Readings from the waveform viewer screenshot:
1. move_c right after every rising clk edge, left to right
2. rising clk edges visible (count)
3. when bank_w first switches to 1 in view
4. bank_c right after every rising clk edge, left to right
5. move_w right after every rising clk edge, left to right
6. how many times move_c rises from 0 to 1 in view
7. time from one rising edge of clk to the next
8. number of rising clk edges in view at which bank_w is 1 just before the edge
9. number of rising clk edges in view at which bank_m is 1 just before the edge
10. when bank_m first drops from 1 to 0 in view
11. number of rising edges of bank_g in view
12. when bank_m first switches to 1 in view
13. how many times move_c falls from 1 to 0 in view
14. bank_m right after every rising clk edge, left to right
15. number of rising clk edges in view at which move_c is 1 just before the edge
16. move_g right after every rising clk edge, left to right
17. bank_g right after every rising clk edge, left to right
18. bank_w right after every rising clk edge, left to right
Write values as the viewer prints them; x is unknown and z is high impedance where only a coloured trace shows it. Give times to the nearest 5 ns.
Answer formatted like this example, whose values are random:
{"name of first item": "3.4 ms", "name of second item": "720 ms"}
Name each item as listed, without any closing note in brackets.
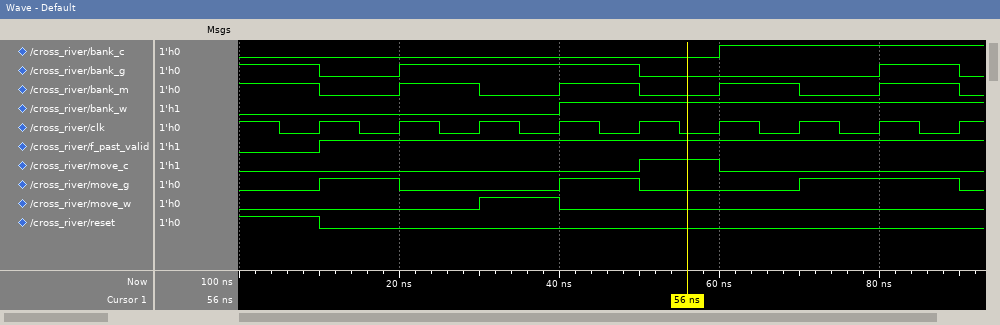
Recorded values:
{"move_c right after every rising clk edge, left to right": "0 0 0 0 1 0 0 0 0", "rising clk edges visible": "9", "when bank_w first switches to 1 in view": "40 ns", "bank_c right after every rising clk edge, left to right": "0 0 0 0 0 1 1 1 1", "move_w right after every rising clk edge, left to right": "0 0 1 0 0 0 0 0 0", "how many times move_c rises from 0 to 1 in view": "1", "time from one rising edge of clk to the next": "10 ns", "number of rising clk edges in view at which bank_w is 1 just before the edge": "5", "number of rising clk edges in view at which bank_m is 1 just before the edge": "5", "when bank_m first drops from 1 to 0 in view": "10 ns", "number of rising edges of bank_g in view": "2", "when bank_m first switches to 1 in view": "20 ns", "how many times move_c falls from 1 to 0 in view": "1", "bank_m right after every rising clk edge, left to right": "0 1 0 1 0 1 0 1 0", "number of rising clk edges in view at which move_c is 1 just before the edge": "1", "move_g right after every rising clk edge, left to right": "1 0 0 1 0 0 1 1 0", "bank_g right after every rising clk edge, left to right": "0 1 1 1 0 0 0 1 0", "bank_w right after every rising clk edge, left to right": "0 0 0 1 1 1 1 1 1"}
